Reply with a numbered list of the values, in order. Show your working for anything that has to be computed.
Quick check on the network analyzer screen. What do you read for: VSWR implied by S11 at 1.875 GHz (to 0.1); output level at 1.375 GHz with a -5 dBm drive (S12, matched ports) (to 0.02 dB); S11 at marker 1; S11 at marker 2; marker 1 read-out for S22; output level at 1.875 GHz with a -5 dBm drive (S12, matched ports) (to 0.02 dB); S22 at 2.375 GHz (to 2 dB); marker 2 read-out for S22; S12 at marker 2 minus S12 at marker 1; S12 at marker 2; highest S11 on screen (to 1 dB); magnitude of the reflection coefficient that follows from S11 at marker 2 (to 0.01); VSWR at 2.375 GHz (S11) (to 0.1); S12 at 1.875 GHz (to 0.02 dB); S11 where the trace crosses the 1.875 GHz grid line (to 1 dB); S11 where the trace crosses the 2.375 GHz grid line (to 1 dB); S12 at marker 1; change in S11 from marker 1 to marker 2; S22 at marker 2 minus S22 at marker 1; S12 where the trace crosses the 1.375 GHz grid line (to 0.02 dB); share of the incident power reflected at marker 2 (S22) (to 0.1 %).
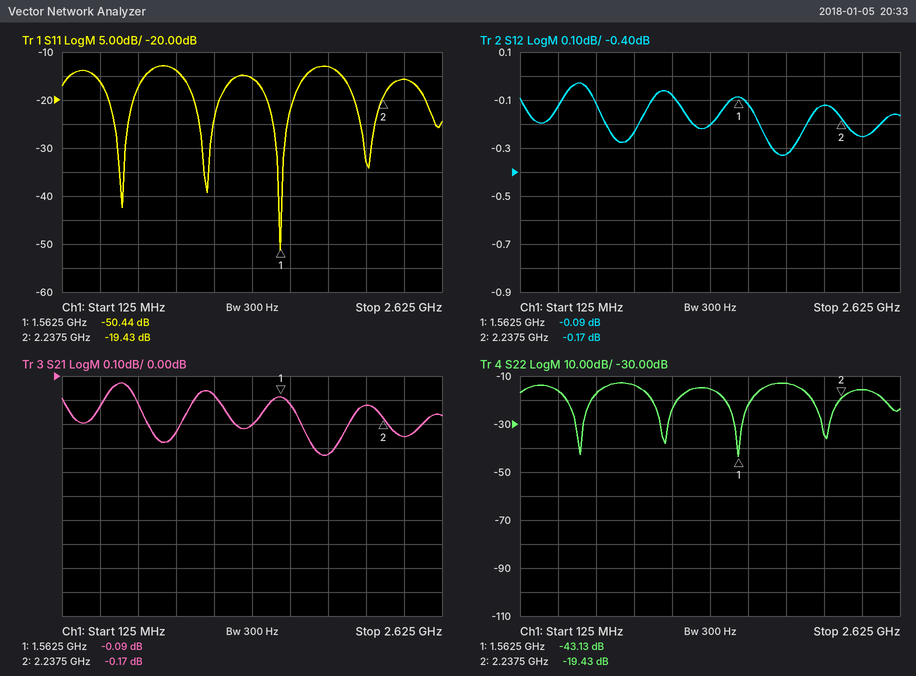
1. |Γ| = 10^(-13/20) = 0.2239; VSWR = (1 + 0.2239)/(1 − 0.2239) ≈ 1.6
2. -5 dBm + (-0.20 dB) = -5.20 dBm
3. -50.44 dB
4. -19.43 dB
5. -43.13 dB
6. -5 dBm + (-0.32 dB) = -5.32 dBm
7. -16 dB
8. -19.43 dB
9. -0.17 − (-0.09) = -0.08 dB
10. -0.17 dB
11. -13 dB
12. 10^(-19.43/20) ≈ 0.11
13. |Γ| = 10^(-16/20) = 0.1585; VSWR = (1 + 0.1585)/(1 − 0.1585) ≈ 1.4
14. -0.32 dB
15. -13 dB
16. -16 dB
17. -0.09 dB
18. -19.43 − (-50.44) = 31.01 dB
19. -19.43 − (-43.13) = 23.70 dB
20. -0.20 dB
21. 10^(-19.43/10) ≈ 1.1 %
